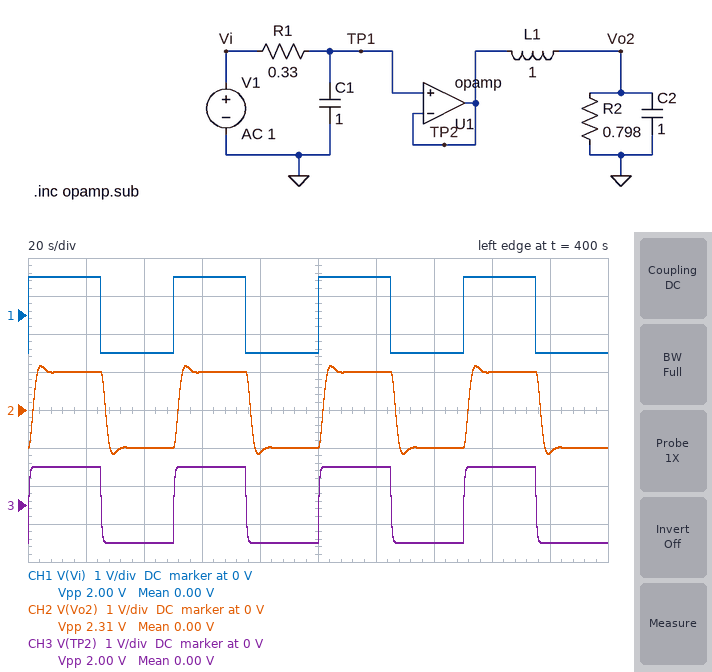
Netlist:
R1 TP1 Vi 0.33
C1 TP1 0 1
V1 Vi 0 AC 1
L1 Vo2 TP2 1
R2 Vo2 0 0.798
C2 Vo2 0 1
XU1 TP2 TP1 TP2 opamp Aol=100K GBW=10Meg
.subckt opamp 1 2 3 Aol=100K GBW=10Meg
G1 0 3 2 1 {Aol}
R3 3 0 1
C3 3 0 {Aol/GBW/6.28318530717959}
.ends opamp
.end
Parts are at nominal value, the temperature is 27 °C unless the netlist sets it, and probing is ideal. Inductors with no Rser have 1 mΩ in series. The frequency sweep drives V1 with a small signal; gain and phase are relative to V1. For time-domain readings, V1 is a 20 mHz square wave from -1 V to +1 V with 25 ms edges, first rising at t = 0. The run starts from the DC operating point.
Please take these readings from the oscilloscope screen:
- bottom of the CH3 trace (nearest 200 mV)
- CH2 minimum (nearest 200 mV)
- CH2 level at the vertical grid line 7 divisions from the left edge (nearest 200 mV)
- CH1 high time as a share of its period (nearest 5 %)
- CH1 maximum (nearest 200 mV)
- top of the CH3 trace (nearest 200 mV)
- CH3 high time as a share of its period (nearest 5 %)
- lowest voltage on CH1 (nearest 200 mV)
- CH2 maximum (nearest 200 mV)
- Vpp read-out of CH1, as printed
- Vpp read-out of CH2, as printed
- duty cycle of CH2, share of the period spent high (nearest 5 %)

-1.0 V
-1.2 V
-1.0 V
50 %
1.0 V
1.0 V
50 %
-1.0 V
1.2 V
2.00 V
2.31 V
50 %
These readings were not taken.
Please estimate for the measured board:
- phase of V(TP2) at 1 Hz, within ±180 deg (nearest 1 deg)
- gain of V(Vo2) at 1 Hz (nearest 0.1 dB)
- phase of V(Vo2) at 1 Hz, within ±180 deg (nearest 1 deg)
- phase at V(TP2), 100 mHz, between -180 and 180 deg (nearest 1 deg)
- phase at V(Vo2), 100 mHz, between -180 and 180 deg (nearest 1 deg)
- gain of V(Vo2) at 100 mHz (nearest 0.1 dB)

-64 deg
-39.1 dB
127 deg
-12 deg
-64 deg
-0.1 dB
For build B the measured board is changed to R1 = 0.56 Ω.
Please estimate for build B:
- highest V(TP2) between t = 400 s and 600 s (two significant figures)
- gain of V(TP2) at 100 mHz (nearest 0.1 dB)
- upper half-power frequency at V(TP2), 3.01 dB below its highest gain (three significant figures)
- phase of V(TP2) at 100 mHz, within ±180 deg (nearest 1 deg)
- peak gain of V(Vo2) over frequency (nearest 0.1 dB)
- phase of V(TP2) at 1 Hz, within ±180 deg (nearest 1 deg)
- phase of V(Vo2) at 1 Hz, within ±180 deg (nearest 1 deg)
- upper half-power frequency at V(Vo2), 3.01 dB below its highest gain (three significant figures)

1.0 V
-0.5 dB
284 mHz
-19 deg
0 dB
-74 deg
117 deg
157 mHz
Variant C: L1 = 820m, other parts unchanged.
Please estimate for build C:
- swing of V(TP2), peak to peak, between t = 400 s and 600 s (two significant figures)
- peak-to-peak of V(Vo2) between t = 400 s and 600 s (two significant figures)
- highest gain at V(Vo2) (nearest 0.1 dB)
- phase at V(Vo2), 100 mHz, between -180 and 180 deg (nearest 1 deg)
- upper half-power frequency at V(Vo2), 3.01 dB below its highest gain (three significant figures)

2.0 V
2.4 V
0.4 dB
-55 deg
192 mHz
